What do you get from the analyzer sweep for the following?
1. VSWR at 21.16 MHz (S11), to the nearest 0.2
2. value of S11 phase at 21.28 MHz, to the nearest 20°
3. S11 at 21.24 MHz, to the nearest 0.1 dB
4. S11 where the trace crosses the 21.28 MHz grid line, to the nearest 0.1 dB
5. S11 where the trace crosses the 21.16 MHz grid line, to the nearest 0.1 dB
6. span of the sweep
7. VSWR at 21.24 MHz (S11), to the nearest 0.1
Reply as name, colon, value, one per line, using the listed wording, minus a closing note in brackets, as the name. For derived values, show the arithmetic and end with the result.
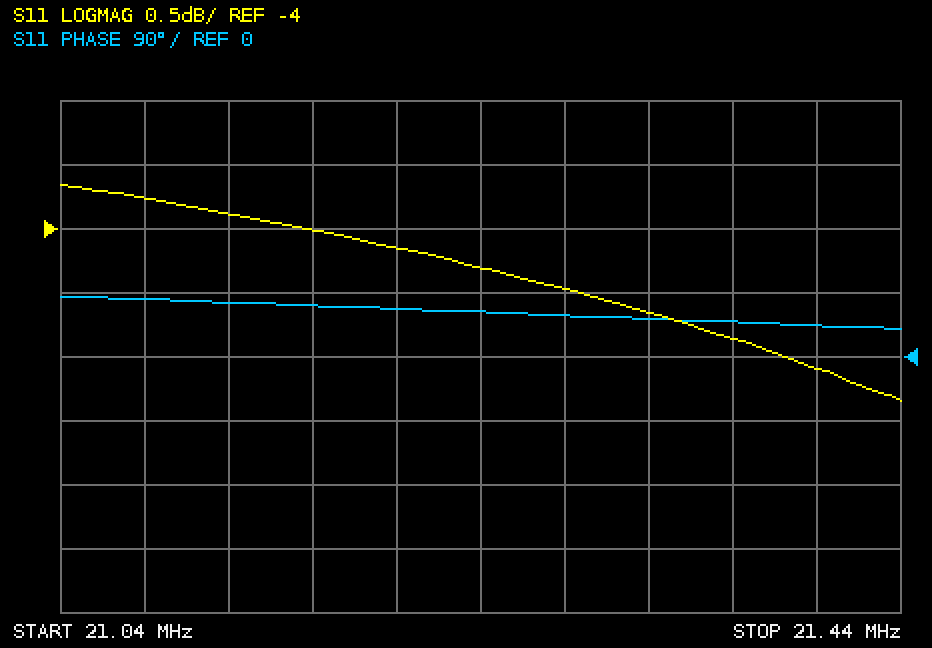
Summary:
VSWR at 21.16 MHz (S11), to the nearest 0.2: |Γ| = 10^(-4/20) = 0.6310; VSWR = (1 + 0.6310)/(1 − 0.6310) ≈ 4.4
value of S11 phase at 21.28 MHz, to the nearest 20°: 60°
S11 at 21.24 MHz, to the nearest 0.1 dB: -4.3 dB
S11 where the trace crosses the 21.28 MHz grid line, to the nearest 0.1 dB: -4.5 dB
S11 where the trace crosses the 21.16 MHz grid line, to the nearest 0.1 dB: -4.0 dB
span of the sweep: 400 kHz
VSWR at 21.24 MHz (S11), to the nearest 0.1: |Γ| = 10^(-4.3/20) = 0.6095; VSWR = (1 + 0.6095)/(1 − 0.6095) ≈ 4.1
